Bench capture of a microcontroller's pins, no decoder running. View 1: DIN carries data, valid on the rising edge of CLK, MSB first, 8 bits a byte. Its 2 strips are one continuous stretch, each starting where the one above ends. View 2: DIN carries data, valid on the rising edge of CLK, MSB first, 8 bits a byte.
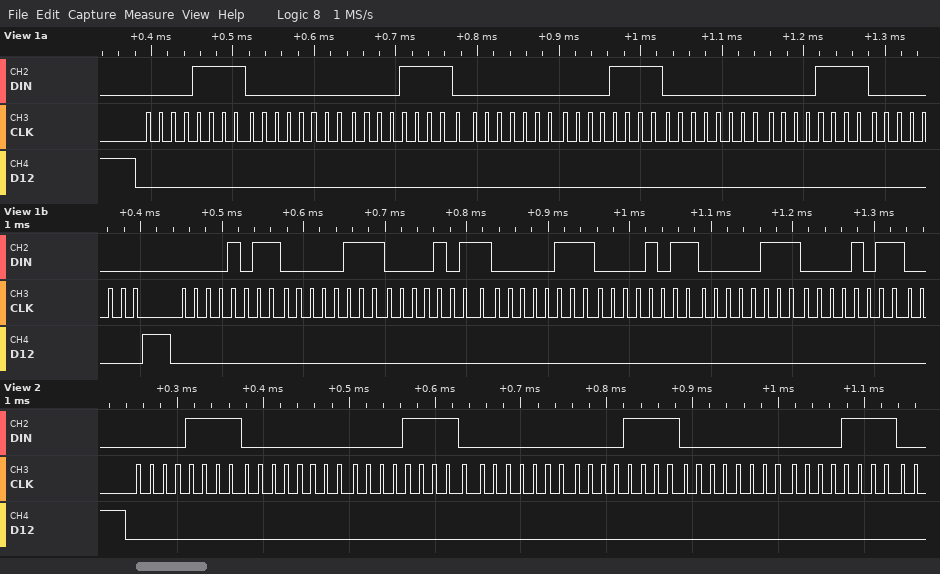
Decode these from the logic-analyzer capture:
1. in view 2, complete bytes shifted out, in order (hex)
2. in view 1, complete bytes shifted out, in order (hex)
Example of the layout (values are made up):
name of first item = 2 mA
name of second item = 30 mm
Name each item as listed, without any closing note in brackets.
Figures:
in view 2, complete bytes shifted out, in order = 0F 00 0F 00 0F 00 0F
in view 1, complete bytes shifted out, in order = 0x0F 0x00 0x0F 0x00 0x0F 0x00 0x0F 0x00 0x0B 0x07 0x0B 0x07 0x0B 0x07 0x0B
